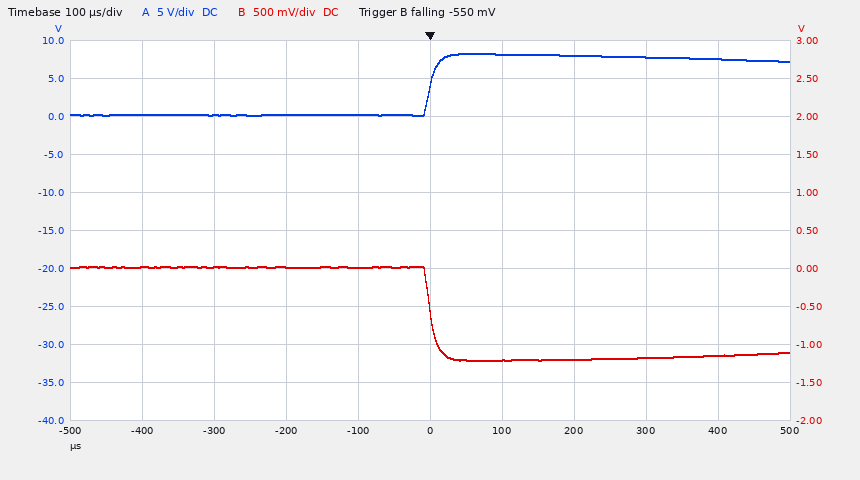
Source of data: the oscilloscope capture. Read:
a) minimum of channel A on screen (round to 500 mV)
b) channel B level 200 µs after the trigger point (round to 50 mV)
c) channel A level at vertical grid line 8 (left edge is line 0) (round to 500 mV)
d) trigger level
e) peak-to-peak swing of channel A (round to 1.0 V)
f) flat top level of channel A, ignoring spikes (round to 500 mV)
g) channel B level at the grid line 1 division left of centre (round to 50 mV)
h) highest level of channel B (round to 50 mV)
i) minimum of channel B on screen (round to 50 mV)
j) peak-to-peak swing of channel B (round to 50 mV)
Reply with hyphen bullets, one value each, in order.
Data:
- 0.0 V
- -1.20 V
- 8.0 V
- -550 mV
- 8.0 V
- 8.0 V
- 0 mV
- 50 mV
- -1.20 V
- 1.25 V
